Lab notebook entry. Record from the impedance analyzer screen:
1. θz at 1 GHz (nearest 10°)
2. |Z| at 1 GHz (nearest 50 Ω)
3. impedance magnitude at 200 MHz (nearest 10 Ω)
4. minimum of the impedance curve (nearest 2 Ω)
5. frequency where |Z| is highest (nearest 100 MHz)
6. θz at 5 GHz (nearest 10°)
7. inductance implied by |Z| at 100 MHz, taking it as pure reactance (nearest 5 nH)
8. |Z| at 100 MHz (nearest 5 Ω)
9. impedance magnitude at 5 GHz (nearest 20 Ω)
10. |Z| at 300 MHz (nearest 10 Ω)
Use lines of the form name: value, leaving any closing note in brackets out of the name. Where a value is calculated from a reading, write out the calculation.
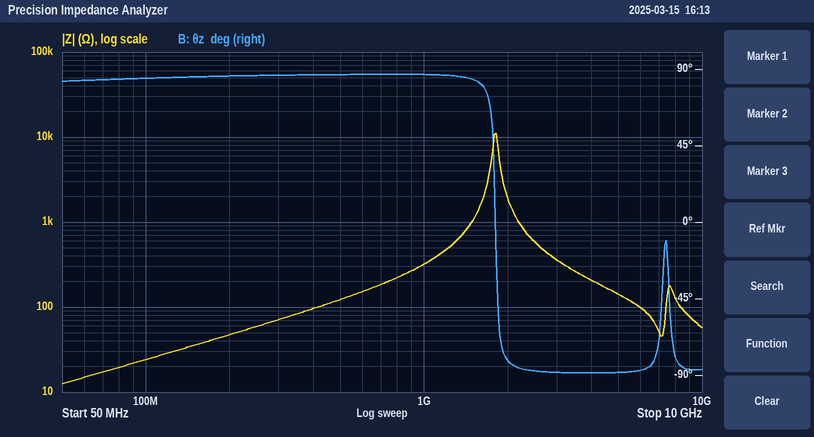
θz at 1 GHz: 90°
|Z| at 1 GHz: 300 Ω
impedance magnitude at 200 MHz: 50 Ω
minimum of the impedance curve: 12 Ω
frequency where |Z| is highest: 1.8 GHz
θz at 5 GHz: -90°
inductance implied by |Z| at 100 MHz, taking it as pure reactance: L = 25 Ω/(2π × 100 MHz) ≈ 40 nH
|Z| at 100 MHz: 25 Ω
impedance magnitude at 5 GHz: 140 Ω
|Z| at 300 MHz: 70 Ω
